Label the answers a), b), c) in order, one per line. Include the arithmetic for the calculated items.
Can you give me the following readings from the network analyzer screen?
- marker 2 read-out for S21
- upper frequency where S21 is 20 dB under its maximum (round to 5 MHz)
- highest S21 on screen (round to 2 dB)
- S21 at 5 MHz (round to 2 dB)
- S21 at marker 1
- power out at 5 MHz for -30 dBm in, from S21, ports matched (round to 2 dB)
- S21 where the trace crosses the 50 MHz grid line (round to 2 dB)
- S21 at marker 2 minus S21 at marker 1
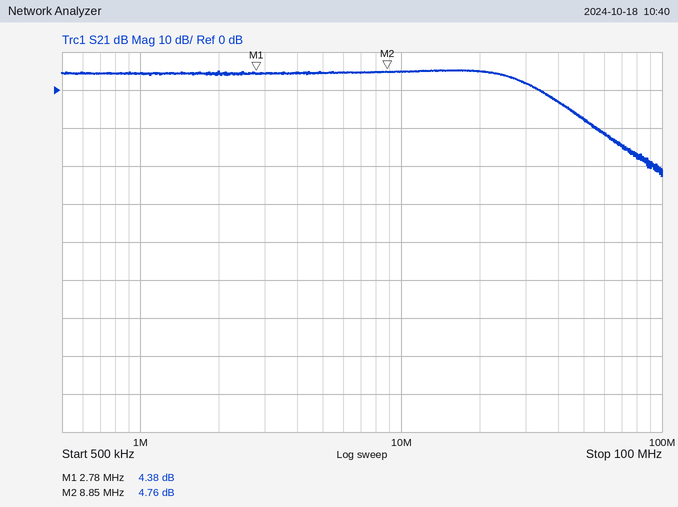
a) 4.76 dB
b) 70 MHz
c) 6 dB
d) 4 dB
e) 4.38 dB
f) -30 dBm + (4 dB) = -26 dBm
g) -8 dB
h) 4.76 − (4.38) = 0.38 dB
